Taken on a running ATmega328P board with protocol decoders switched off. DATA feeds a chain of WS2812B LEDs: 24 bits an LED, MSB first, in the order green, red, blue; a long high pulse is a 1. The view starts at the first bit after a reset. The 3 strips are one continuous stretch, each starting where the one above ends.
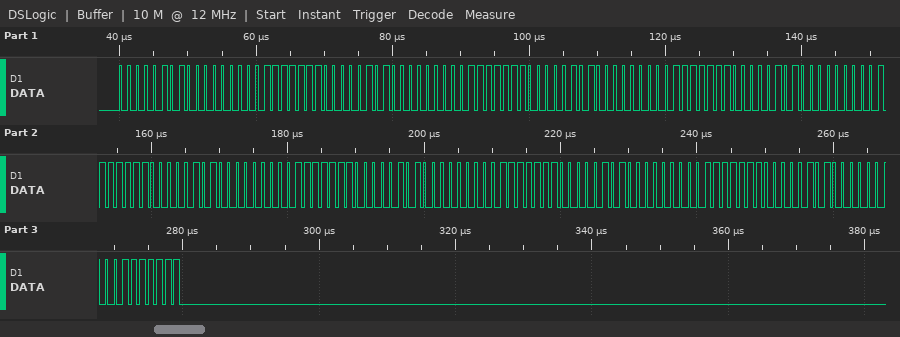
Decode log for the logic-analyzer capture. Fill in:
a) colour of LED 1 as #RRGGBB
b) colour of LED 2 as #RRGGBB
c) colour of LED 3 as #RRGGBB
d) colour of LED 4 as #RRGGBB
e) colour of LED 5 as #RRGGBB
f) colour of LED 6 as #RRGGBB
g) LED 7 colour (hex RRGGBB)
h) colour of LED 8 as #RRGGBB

#00057F
#00057F
#00057F
#00057F
#00057F
#00057F
#00057F
#00057F
